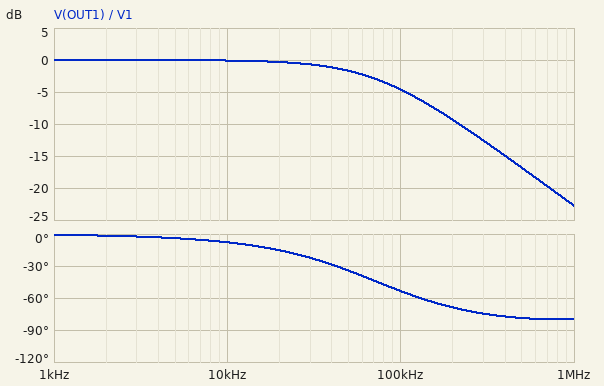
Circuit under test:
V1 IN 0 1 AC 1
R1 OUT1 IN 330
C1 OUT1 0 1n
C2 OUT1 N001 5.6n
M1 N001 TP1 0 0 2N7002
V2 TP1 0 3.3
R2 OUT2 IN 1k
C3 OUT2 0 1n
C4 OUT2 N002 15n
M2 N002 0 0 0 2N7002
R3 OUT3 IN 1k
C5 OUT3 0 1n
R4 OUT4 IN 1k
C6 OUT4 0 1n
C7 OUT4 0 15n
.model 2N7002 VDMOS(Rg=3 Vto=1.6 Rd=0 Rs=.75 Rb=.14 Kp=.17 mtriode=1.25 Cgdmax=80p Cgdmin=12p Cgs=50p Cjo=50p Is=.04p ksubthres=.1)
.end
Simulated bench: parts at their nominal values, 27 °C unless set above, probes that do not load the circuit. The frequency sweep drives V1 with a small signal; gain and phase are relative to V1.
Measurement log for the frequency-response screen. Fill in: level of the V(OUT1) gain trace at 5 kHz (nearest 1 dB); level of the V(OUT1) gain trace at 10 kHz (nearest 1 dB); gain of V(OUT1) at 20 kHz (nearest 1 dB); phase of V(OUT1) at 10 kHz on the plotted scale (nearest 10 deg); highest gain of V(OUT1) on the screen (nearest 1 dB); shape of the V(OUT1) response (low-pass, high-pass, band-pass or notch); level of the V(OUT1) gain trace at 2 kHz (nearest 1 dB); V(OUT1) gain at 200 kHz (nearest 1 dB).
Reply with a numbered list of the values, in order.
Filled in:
1. 0 dB
2. 0 dB
3. 0 dB
4. -10 deg
5. 0 dB
6. low-pass
7. 0 dB
8. -9 dB
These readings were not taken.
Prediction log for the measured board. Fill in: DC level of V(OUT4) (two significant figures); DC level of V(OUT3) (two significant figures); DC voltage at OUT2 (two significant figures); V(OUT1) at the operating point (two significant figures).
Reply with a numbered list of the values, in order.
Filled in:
1. 1.0 V
2. 1.0 V
3. 1.0 V
4. 1.0 V
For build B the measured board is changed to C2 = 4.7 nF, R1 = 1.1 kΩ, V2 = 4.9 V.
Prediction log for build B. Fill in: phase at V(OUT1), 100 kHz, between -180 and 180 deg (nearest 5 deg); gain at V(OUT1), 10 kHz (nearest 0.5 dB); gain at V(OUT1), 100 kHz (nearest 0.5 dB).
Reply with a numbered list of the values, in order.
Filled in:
1. -75 deg
2. -0.5 dB
3. -12.0 dB
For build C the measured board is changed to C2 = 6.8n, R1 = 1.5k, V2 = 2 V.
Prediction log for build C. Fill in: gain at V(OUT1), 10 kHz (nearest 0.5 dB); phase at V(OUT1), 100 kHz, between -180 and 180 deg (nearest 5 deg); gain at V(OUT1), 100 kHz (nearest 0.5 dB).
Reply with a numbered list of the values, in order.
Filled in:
1. -2.0 dB
2. -80 deg
3. -17.5 dB
